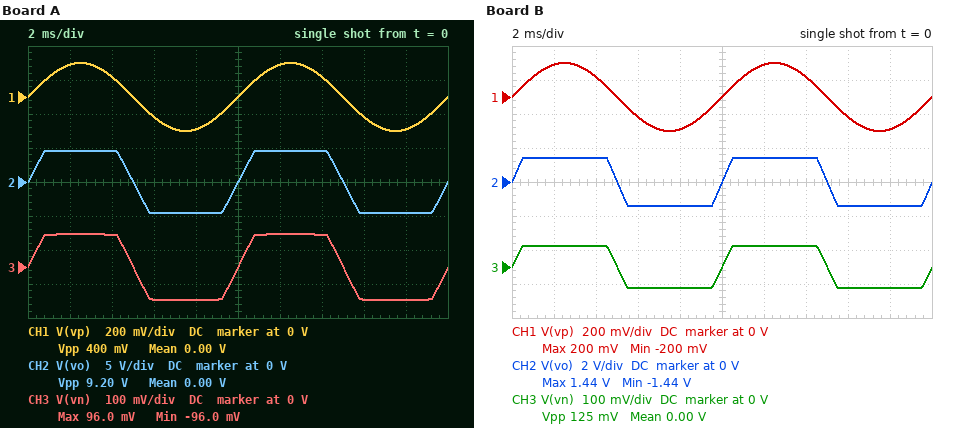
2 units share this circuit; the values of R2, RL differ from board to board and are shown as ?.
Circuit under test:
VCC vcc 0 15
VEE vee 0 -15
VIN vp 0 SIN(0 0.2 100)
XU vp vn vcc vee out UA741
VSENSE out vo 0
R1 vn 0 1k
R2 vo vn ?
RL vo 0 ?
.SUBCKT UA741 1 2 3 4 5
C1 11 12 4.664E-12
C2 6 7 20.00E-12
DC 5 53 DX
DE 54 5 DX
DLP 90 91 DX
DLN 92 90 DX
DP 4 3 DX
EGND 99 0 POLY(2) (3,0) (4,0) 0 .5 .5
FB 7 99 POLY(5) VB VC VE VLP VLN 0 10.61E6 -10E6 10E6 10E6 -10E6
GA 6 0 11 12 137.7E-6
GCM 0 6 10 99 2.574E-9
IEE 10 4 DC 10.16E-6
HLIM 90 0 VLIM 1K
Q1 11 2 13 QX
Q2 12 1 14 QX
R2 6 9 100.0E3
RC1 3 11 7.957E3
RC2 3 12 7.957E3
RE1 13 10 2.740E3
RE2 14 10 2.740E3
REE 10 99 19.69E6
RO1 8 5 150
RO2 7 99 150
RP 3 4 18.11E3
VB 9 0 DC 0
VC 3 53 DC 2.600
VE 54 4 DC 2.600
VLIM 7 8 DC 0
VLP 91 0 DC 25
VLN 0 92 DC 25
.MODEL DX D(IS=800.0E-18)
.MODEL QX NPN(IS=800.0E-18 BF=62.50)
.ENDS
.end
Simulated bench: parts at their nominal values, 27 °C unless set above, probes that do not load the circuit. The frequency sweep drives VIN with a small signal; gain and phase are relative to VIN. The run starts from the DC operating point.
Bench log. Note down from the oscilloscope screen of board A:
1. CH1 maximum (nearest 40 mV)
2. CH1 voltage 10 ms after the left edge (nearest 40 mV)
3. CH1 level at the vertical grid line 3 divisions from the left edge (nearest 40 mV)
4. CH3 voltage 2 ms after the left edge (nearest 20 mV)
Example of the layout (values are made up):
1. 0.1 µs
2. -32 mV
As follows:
1. 200 mV
2. 0 V
3. -120 mV
4. 100 mV
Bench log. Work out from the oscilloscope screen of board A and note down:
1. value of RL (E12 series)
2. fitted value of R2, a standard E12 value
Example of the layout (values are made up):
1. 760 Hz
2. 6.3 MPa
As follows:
1. 180 Ω
2. 47 kΩ
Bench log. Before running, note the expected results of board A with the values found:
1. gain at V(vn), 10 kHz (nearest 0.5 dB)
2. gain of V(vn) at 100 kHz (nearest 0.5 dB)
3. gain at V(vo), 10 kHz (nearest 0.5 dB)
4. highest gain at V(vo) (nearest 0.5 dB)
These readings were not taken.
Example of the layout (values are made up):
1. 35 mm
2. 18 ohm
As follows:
1. -2.0 dB
2. -18.0 dB
3. 31.5 dB
4. 33.5 dB
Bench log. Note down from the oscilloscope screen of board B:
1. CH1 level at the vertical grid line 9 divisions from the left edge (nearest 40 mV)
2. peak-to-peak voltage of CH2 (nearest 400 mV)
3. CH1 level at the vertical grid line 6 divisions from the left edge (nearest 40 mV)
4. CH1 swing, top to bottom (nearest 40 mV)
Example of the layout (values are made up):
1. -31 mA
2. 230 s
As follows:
1. -200 mV
2. 2.8 V
3. 200 mV
4. 400 mV
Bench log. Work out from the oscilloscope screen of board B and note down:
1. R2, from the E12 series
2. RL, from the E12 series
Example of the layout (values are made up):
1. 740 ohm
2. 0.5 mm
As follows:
1. 22 kΩ
2. 56 Ω
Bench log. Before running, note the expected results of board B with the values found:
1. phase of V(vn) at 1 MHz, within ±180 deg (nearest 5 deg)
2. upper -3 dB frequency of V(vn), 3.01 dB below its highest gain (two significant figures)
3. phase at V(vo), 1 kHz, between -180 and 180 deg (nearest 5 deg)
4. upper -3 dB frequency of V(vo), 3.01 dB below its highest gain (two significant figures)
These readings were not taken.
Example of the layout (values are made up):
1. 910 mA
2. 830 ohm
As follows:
1. -110 deg
2. 13 kHz
3. -5 deg
4. 13 kHz
